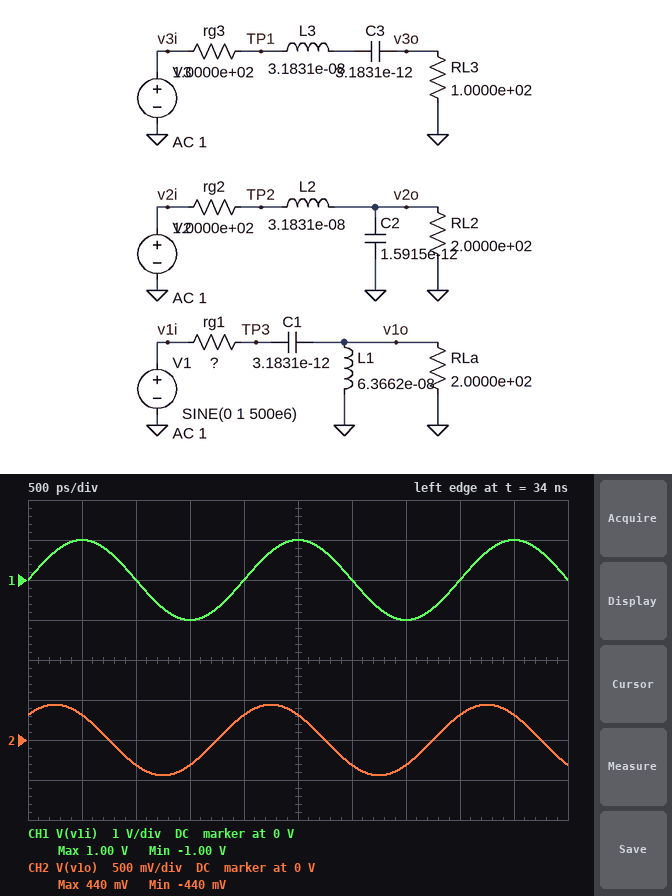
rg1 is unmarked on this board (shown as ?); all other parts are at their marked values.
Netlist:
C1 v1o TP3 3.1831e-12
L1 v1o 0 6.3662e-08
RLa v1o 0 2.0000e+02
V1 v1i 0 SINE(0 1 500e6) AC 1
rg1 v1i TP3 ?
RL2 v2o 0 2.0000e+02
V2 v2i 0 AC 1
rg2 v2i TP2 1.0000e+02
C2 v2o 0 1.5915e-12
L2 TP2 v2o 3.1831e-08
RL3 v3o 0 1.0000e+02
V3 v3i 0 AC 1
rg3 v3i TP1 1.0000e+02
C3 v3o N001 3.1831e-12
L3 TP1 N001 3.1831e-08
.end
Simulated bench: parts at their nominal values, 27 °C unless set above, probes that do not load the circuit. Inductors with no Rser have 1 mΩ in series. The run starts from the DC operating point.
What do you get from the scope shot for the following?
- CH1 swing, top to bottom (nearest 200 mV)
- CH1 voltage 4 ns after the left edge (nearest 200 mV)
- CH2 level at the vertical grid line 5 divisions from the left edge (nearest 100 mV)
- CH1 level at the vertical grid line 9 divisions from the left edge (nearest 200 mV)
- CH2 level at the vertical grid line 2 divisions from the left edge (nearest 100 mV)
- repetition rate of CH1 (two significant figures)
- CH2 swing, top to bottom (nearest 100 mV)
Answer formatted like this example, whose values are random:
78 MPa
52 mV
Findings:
2.0 V
0 V
300 mV
1.0 V
-300 mV
500 MHz
900 mV
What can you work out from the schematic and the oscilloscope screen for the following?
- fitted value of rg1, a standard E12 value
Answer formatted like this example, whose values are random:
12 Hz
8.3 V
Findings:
220 Ω
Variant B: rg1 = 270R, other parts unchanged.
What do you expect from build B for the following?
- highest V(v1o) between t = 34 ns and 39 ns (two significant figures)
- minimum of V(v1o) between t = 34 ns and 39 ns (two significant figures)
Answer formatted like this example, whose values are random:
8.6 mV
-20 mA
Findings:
380 mV
-380 mV
